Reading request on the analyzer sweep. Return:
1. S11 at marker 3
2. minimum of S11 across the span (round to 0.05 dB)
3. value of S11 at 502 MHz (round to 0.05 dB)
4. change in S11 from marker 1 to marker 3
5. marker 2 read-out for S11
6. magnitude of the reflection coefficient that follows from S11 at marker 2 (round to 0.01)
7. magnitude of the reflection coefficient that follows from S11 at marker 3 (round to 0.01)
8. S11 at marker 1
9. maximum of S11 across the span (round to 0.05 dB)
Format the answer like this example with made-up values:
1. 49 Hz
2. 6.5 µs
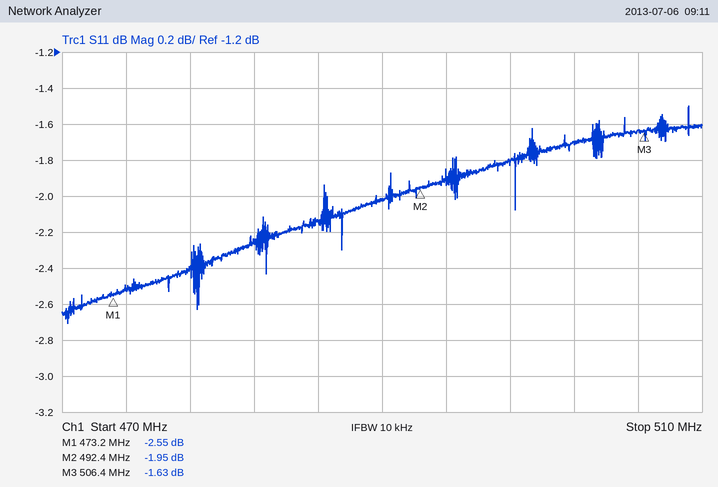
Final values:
1. -1.63 dB
2. -2.70 dB
3. -1.70 dB
4. 0.92 dB
5. -1.95 dB
6. 0.80
7. 0.83
8. -2.55 dB
9. -1.50 dB
